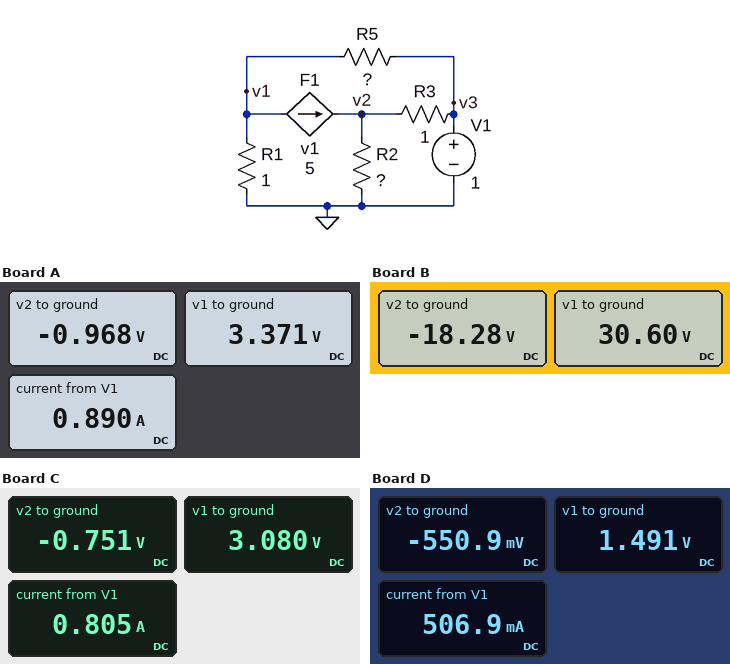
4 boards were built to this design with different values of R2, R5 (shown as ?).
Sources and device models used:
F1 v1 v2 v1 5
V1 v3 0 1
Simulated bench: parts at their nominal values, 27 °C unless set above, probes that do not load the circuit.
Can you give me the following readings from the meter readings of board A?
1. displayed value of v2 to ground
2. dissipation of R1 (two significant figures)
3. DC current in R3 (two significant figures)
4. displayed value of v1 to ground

-0.968 V
11 W
2.0 A
3.371 V
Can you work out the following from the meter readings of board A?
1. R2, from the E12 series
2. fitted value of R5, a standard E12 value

0.39 Ω
2.2 Ω
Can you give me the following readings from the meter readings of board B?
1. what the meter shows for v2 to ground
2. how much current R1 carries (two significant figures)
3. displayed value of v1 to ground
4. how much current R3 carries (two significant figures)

-18.28 V
31 A
30.60 V
19 A
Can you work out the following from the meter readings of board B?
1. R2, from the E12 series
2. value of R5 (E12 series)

0.82 Ω
2.7 Ω
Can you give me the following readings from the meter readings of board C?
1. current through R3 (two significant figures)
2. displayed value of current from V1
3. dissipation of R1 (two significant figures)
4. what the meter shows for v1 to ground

1.8 A
0.805 A
9.5 W
3.080 V
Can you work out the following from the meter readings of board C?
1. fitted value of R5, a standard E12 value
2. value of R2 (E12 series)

2.2 Ω
0.33 Ω
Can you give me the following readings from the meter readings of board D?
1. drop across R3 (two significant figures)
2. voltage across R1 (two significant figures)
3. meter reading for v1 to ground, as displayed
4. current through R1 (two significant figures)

1.6 V
1.5 V
1.491 V
1.5 A
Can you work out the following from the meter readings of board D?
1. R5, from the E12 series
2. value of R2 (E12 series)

0.47 Ω
0.56 Ω
